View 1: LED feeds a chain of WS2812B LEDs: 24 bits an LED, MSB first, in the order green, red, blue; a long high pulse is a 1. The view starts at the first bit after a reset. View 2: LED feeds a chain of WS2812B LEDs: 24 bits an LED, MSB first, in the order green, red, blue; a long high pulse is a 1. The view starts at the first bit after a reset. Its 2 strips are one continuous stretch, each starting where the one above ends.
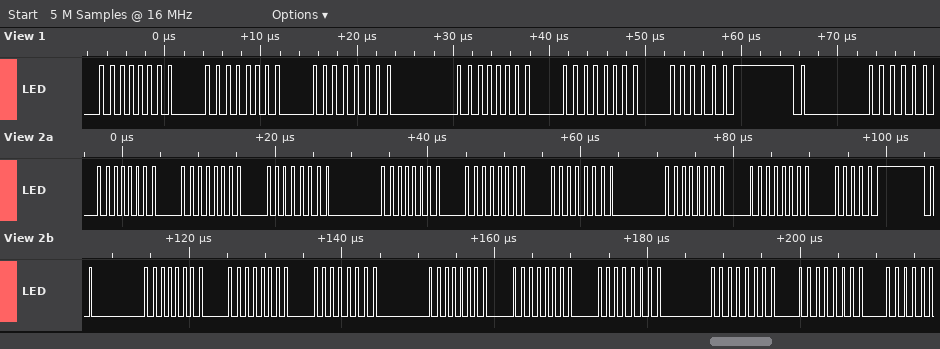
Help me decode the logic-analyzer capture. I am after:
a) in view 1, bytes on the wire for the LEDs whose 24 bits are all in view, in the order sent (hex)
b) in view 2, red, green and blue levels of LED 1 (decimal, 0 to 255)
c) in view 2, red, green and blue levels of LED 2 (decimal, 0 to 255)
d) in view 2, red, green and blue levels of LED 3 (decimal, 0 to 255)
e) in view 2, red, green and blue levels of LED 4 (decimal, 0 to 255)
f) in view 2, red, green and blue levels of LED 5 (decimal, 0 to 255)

00 00 00 00 00 02
0, 0, 0
0, 0, 0
0, 0, 4
0, 0, 0
0, 0, 0
